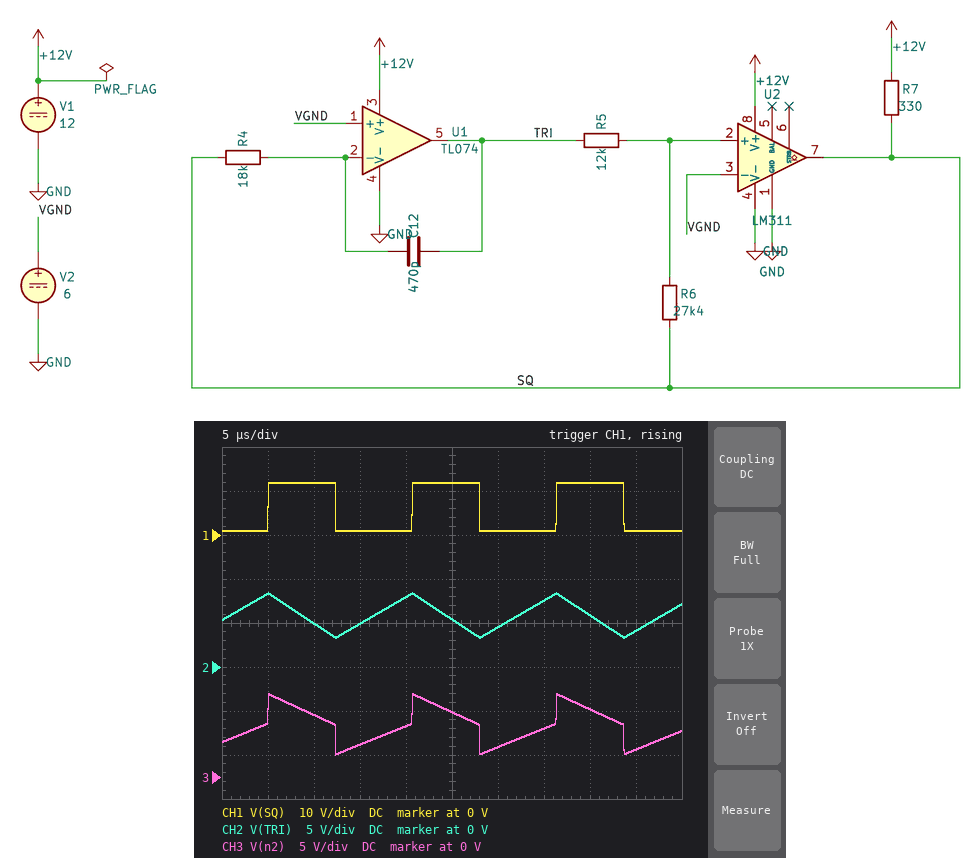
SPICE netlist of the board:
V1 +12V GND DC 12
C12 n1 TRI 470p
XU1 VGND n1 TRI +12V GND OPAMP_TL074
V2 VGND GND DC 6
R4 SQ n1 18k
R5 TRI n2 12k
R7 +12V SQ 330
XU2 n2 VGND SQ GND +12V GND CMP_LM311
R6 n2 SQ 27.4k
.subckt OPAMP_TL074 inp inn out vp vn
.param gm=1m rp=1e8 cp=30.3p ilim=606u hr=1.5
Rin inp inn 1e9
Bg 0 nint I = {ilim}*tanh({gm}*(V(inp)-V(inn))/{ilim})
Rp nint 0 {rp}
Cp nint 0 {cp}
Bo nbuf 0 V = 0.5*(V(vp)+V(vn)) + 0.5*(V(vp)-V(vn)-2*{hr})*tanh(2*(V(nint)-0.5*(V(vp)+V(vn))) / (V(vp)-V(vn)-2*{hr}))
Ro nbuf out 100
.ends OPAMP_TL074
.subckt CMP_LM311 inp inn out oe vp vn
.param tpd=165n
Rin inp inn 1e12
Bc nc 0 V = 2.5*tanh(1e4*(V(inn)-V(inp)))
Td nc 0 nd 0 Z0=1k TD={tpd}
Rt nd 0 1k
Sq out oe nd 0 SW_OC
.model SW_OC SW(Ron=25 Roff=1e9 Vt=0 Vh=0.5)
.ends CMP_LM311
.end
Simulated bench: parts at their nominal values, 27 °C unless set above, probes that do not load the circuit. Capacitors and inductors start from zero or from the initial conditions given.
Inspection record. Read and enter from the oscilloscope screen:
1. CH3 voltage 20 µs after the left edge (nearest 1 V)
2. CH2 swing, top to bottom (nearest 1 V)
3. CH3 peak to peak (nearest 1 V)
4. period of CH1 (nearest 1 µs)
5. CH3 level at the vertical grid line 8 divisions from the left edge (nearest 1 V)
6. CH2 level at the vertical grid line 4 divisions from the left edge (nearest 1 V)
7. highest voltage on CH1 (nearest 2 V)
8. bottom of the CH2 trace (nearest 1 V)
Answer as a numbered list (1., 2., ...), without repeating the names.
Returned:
1. 6 V
2. 5 V
3. 7 V
4. 16 µs
5. 8 V
6. 8 V
7. 12 V
8. 3 V
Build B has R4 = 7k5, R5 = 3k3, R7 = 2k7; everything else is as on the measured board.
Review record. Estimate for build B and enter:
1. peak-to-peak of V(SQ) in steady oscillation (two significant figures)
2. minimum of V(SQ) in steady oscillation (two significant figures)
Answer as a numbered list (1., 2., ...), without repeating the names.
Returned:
1. 10 V
2. 130 mV
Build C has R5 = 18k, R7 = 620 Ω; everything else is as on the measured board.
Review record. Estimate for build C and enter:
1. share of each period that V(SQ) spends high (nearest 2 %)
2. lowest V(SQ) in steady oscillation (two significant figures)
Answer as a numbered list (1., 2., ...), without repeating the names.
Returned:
1. 50 %
2. 470 mV
